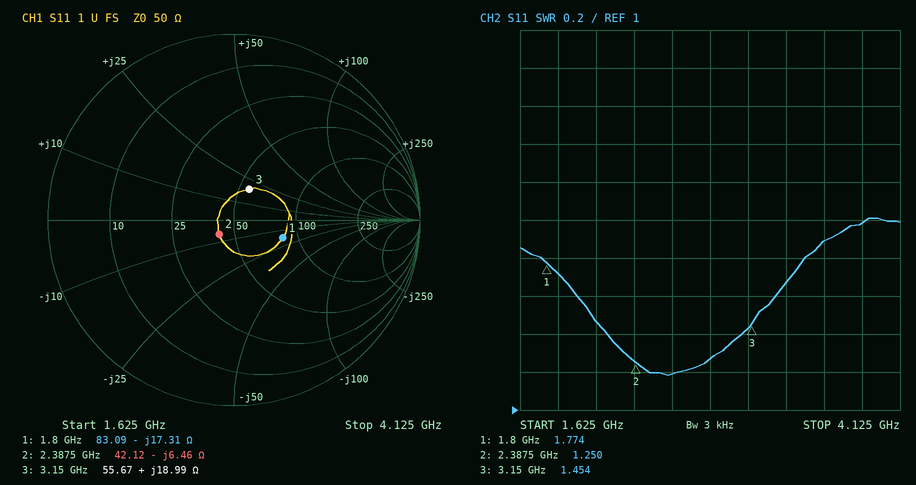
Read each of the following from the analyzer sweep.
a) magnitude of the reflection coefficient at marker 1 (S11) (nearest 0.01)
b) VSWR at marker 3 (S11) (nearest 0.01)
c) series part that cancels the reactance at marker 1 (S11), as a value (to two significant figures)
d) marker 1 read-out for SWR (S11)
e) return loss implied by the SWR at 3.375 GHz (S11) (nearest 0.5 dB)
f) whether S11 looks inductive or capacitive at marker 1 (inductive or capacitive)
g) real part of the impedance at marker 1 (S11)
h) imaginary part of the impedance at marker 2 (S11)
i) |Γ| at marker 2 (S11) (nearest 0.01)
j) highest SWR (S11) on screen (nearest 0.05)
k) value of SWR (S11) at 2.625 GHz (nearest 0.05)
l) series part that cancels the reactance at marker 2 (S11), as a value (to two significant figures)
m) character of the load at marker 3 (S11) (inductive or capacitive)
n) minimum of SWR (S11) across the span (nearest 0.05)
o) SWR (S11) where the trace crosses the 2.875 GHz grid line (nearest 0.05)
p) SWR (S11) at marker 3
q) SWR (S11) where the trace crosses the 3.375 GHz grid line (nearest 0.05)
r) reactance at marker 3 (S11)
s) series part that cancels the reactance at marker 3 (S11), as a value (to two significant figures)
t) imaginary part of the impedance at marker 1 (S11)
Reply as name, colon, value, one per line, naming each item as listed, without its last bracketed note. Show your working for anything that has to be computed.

magnitude of the reflection coefficient at marker 1 (S11): 0.28
VSWR at marker 3 (S11): 1.45
series part that cancels the reactance at marker 1 (S11), as a value: L = 17.31 Ω/(2π × 1.8 GHz) ≈ 1.5 nH
marker 1 read-out for SWR: 1.774
return loss implied by the SWR at 3.375 GHz (S11): −20 log10((1.65 − 1)/(1.65 + 1)) ≈ 12.2 dB, so 12.0 dB to the nearest 0.5 dB
whether S11 looks inductive or capacitive at marker 1: capacitive
real part of the impedance at marker 1: 83.09 Ω
imaginary part of the impedance at marker 2: -6.46 Ω
|Γ| at marker 2 (S11): 0.11
highest SWR (S11) on screen: 2.00
value of SWR (S11) at 2.625 GHz: 1.20
series part that cancels the reactance at marker 2 (S11), as a value: L = 6.46 Ω/(2π × 2.3875 GHz) ≈ 431 pH, so 430 pH to two significant figures
character of the load at marker 3 (S11): inductive
minimum of SWR (S11) across the span: 1.20
SWR (S11) where the trace crosses the 2.875 GHz grid line: 1.25
SWR (S11) at marker 3: 1.454
SWR (S11) where the trace crosses the 3.375 GHz grid line: 1.65
reactance at marker 3: +18.99 Ω
series part that cancels the reactance at marker 3 (S11), as a value: C = 1/(2π × 3.15 GHz × 18.99 Ω) ≈ 2.7 pF
imaginary part of the impedance at marker 1: -17.31 Ω
